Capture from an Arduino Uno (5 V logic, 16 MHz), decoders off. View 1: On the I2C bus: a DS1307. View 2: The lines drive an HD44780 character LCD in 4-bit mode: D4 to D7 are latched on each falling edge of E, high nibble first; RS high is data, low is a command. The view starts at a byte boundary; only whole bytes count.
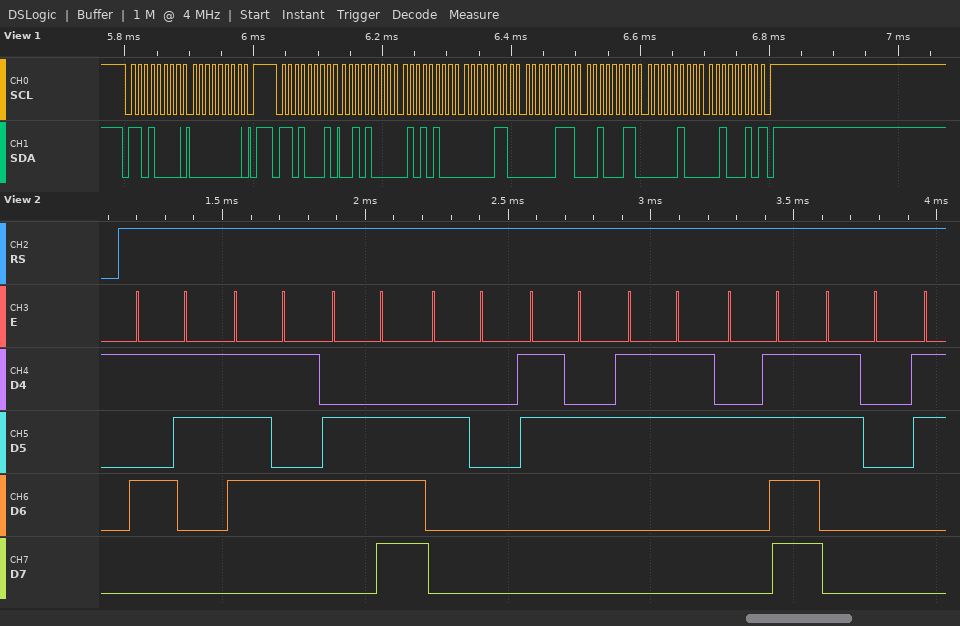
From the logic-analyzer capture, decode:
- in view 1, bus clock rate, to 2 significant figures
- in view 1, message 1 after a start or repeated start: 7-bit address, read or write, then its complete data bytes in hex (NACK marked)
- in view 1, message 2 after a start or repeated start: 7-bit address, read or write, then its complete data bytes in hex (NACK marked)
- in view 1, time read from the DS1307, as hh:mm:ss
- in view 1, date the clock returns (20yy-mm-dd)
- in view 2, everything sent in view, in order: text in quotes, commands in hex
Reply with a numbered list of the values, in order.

1. 100 kHz
2. 0x68 write: 00
3. 0x68 read: 28 54 06 07 23 04 22 NACK
4. 06:54:28
5. 2022-04-23
6. "Sun 23/0"
